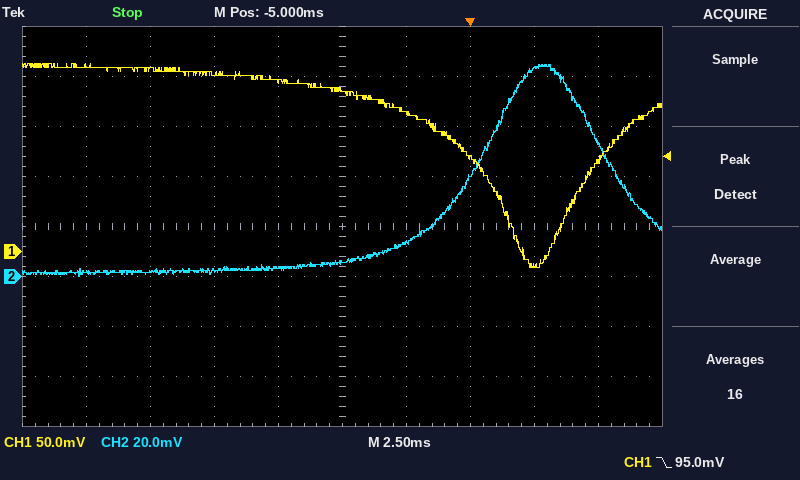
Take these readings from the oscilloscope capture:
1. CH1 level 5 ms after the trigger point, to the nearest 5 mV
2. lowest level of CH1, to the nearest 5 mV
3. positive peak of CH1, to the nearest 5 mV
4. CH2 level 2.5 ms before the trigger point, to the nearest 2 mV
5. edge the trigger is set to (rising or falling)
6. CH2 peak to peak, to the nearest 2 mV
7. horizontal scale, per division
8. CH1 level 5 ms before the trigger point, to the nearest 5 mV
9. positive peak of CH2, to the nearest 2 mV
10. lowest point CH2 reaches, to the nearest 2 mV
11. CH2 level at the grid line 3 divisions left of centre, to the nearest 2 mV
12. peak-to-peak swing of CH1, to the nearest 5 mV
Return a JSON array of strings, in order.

["90 mV", "-15 mV", "190 mV", "14 mV", "falling", "84 mV", "2.5 ms", "160 mV", "84 mV", "0 mV", "2 mV", "205 mV"]
